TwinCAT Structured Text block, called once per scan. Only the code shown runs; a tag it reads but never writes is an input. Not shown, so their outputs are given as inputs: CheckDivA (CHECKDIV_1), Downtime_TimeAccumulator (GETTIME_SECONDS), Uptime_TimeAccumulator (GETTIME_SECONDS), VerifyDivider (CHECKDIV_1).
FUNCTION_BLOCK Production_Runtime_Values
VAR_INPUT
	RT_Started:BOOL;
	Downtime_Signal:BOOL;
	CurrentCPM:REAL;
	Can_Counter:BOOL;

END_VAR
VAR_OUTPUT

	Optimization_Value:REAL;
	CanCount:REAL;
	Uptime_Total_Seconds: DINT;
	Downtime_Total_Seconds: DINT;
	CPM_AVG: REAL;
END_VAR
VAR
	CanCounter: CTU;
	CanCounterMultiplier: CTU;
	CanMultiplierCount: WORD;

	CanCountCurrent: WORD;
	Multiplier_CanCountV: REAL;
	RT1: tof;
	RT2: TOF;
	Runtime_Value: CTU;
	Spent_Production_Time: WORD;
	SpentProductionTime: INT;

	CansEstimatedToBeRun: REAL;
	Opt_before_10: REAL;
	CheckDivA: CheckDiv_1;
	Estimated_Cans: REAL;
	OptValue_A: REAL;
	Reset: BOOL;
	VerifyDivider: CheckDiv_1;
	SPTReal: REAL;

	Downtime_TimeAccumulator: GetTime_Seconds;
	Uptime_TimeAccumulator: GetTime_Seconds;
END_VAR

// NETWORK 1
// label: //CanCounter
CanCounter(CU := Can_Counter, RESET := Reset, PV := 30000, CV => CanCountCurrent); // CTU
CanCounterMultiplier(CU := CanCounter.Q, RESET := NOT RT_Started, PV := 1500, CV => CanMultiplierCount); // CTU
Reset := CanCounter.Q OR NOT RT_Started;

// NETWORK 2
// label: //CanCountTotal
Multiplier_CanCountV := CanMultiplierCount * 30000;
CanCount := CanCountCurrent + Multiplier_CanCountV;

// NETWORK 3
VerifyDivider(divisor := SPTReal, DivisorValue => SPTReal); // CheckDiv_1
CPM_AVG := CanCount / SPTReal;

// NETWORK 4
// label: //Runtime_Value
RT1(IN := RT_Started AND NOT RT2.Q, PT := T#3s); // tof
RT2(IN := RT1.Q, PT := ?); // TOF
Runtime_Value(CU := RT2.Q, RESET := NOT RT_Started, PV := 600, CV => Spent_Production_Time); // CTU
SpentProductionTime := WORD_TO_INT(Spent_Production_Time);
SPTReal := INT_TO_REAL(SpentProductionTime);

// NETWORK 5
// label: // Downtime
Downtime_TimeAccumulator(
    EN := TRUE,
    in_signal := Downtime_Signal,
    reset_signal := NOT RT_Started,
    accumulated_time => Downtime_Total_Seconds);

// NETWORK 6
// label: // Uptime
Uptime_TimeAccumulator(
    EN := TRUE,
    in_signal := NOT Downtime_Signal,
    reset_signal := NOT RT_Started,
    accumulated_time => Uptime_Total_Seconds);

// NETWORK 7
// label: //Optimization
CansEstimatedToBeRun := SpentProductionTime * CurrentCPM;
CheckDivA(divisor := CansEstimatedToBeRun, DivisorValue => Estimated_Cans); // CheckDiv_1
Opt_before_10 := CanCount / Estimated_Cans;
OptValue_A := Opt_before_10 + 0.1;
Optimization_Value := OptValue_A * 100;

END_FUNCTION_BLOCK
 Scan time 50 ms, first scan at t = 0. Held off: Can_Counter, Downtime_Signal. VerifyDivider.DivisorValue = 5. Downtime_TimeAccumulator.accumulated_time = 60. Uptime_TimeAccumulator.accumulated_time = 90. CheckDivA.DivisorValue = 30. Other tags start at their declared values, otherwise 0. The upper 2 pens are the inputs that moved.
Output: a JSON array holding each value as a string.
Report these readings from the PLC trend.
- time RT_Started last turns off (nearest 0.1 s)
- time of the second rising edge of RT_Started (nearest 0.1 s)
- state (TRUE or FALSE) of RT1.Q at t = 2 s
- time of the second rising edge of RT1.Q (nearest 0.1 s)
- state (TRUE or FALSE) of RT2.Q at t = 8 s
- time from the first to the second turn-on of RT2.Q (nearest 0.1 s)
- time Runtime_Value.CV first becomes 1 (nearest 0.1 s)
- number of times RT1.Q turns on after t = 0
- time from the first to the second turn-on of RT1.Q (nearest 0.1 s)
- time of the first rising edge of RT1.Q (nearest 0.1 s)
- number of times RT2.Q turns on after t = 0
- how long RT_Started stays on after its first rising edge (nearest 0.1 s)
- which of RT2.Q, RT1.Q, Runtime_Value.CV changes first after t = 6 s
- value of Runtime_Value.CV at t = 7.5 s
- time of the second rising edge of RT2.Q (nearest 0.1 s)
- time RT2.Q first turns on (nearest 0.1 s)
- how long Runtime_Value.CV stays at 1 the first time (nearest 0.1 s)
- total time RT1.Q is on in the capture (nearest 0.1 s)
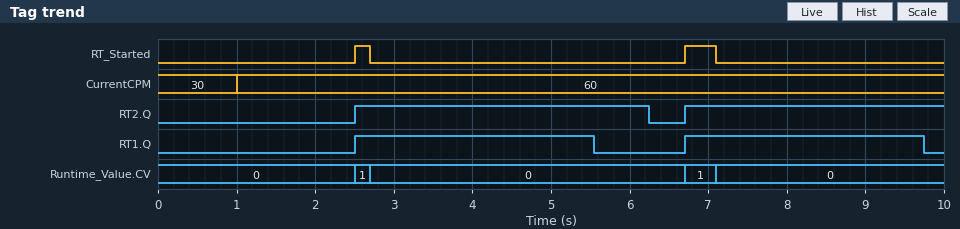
["7.1 s", "6.7 s", "FALSE", "6.7 s", "TRUE", "4.2 s", "2.5 s", "2", "4.2 s", "2.5 s", "2", "0.2 s", "RT2.Q", "0", "6.7 s", "2.5 s", "0.2 s", "6.1 s"]
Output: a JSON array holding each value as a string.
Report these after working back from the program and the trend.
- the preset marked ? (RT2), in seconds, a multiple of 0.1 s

["0.7 s"]
